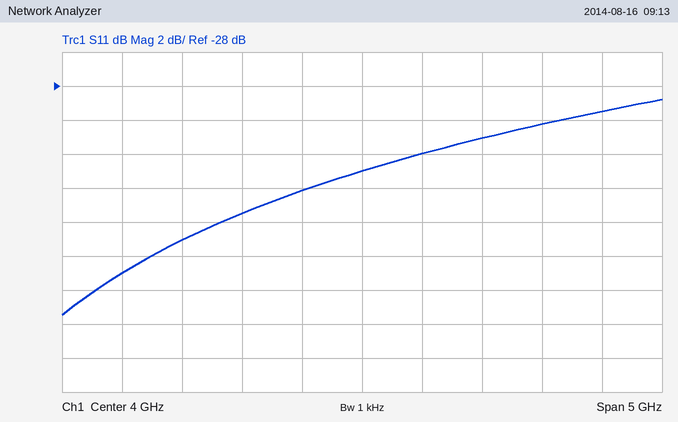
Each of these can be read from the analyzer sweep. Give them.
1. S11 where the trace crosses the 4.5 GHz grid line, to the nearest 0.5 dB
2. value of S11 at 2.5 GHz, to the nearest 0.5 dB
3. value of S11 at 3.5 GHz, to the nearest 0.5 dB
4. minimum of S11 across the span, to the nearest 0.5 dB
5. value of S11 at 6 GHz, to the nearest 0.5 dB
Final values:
-32.0 dB
-37.0 dB
-34.0 dB
-41.5 dB
-29.5 dB
